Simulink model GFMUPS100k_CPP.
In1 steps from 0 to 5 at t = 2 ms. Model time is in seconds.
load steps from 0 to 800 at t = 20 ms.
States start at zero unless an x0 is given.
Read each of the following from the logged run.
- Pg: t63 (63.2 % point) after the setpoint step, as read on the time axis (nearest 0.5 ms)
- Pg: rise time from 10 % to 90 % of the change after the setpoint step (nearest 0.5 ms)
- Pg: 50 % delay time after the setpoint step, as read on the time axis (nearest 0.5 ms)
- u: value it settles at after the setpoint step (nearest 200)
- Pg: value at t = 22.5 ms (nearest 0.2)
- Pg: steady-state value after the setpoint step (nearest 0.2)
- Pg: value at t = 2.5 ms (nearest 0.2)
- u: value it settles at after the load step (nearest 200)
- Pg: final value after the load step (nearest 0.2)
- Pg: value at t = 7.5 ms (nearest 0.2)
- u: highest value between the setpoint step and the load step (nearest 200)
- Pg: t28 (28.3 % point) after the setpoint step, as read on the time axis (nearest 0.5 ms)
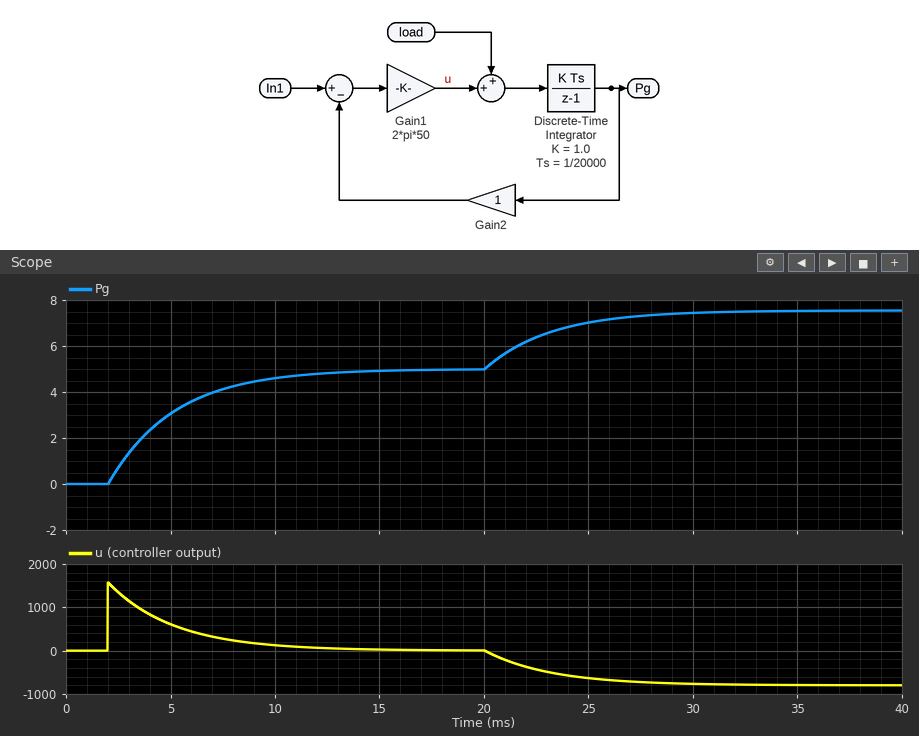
5.0 ms
7.0 ms
4.0 ms
0
6.4
5.0
0.8
-800
7.6
4.2
1600
3.0 ms
